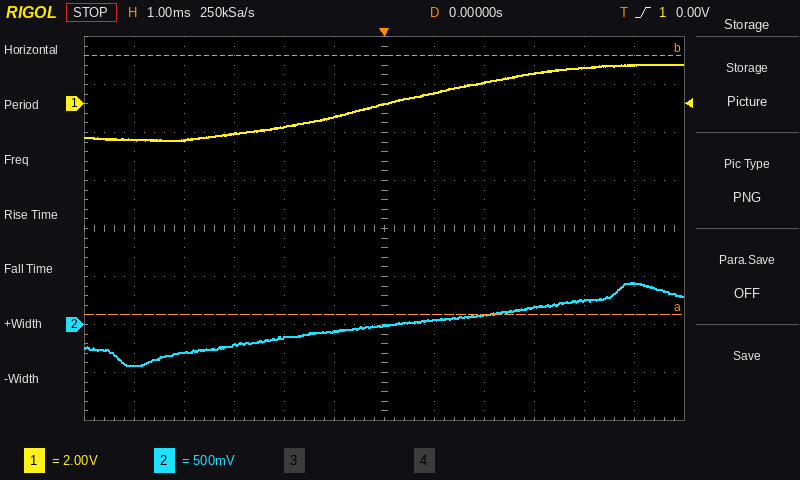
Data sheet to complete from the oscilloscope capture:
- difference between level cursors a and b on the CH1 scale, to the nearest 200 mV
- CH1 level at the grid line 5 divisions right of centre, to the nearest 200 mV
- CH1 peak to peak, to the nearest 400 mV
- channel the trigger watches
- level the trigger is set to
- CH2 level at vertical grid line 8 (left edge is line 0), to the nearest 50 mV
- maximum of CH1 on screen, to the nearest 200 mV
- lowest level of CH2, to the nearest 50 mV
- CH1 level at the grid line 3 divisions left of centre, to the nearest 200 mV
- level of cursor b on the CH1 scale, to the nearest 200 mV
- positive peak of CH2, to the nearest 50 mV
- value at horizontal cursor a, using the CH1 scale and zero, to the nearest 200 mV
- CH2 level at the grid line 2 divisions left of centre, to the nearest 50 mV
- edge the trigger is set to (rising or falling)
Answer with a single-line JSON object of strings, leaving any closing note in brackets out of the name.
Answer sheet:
{"difference between level cursors a and b on the CH1 scale, to the nearest 200 mV": "10.8 V", "CH1 level at the grid line 5 divisions right of centre, to the nearest 200 mV": "1.6 V", "CH1 peak to peak, to the nearest 400 mV": "3.2 V", "channel the trigger watches": "CH1", "level the trigger is set to": "0.00 V", "CH2 level at vertical grid line 8 (left edge is line 0), to the nearest 50 mV": "100 mV", "maximum of CH1 on screen, to the nearest 200 mV": "1.6 V", "lowest level of CH2, to the nearest 50 mV": "-450 mV", "CH1 level at the grid line 3 divisions left of centre, to the nearest 200 mV": "-1.2 V", "level of cursor b on the CH1 scale, to the nearest 200 mV": "2.0 V", "positive peak of CH2, to the nearest 50 mV": "450 mV", "value at horizontal cursor a, using the CH1 scale and zero, to the nearest 200 mV": "-8.8 V", "CH2 level at the grid line 2 divisions left of centre, to the nearest 50 mV": "-150 mV", "edge the trigger is set to": "rising"}
